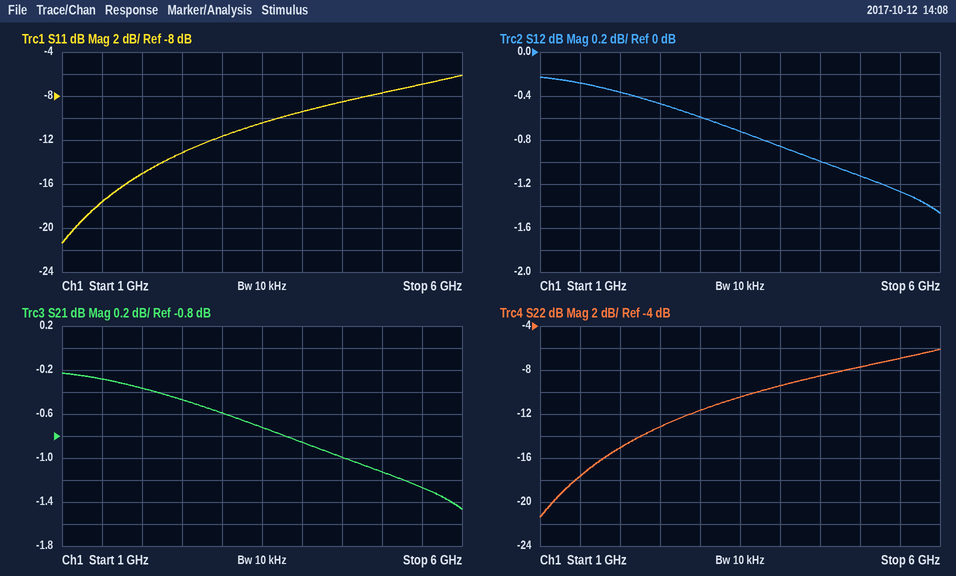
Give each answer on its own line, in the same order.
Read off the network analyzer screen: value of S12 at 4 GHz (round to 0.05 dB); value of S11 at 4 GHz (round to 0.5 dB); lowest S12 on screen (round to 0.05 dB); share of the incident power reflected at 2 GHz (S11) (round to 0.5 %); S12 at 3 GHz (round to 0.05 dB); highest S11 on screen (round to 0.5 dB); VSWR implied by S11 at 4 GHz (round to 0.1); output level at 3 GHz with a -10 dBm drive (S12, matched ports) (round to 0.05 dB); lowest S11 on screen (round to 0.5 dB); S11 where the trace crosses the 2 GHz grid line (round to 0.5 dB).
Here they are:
-0.85 dB
-9.5 dB
-1.45 dB
3.0 %
-0.60 dB
-6.0 dB
2.0
-10.60 dBm
-21.5 dB
-15.0 dB
